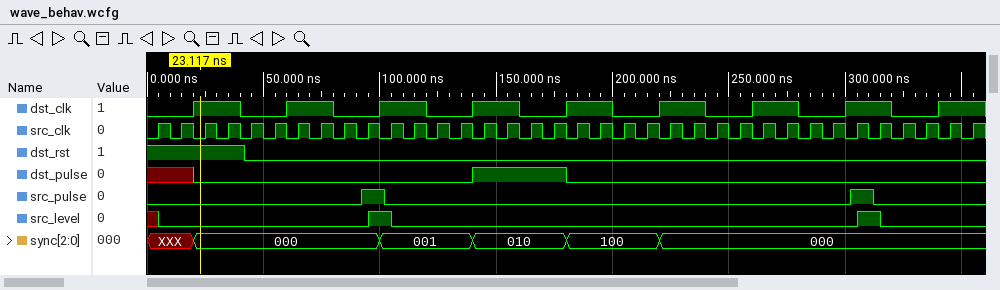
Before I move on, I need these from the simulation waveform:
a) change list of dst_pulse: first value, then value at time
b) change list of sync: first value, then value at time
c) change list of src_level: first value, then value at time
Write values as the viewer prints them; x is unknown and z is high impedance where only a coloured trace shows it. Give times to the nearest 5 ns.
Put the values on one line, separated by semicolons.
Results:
x, 0 at 20 ns, 1 at 140 ns, 0 at 180 ns; XXX, 000 at 20 ns, 001 at 100 ns, 010 at 140 ns, 100 at 180 ns, 000 at 220 ns; x, 0 at 5 ns, 1 at 95 ns, 0 at 105 ns, 1 at 305 ns, 0 at 315 ns
